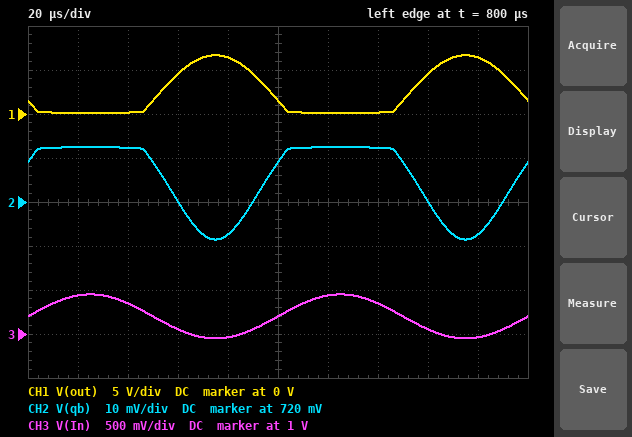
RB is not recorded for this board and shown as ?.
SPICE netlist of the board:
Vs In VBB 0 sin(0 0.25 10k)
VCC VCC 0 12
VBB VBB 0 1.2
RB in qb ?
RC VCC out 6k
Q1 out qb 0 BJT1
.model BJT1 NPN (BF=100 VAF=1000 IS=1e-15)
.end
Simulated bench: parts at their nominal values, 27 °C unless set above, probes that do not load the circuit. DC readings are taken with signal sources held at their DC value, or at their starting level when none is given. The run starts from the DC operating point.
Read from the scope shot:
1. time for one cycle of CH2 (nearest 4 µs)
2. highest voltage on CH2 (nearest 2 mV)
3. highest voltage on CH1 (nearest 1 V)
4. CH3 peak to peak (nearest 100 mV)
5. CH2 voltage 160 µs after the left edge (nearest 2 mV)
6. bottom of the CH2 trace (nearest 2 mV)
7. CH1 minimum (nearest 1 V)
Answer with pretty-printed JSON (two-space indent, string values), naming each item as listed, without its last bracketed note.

{
  "time for one cycle of CH2": "100 µs",
  "highest voltage on CH2": "732 mV",
  "highest voltage on CH1": "7 V",
  "CH3 peak to peak": "500 mV",
  "CH2 voltage 160 µs after the left edge": "720 mV",
  "bottom of the CH2 trace": "712 mV",
  "CH1 minimum": "0 V"
}
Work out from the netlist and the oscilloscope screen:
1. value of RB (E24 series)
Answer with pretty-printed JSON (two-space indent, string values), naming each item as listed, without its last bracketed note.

{
  "value of RB": "27 kΩ"
}
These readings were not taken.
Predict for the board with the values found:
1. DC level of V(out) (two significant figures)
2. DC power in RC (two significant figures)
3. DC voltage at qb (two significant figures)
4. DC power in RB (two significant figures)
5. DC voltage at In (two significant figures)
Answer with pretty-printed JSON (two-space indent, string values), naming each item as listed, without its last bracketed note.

{
  "DC level of V(out)": "1.5 V",
  "DC power in RC": "18 mW",
  "DC voltage at qb": "730 mV",
  "DC power in RB": "8.2 µW",
  "DC voltage at In": "1.2 V"
}
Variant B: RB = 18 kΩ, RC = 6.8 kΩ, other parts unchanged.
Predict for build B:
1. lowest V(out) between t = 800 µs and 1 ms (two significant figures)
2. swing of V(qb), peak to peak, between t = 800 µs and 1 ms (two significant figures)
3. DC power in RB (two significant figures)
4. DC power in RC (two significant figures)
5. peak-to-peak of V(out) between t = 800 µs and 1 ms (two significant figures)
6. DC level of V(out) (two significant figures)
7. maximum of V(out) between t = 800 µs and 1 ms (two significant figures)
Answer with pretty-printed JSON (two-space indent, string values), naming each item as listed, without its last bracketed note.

{
  "lowest V(out) between t = 800 µs and 1 ms": "110 mV",
  "swing of V(qb), peak to peak, between t = 800 µs and 1 ms": "8.9 mV",
  "DC power in RB": "12 µW",
  "DC power in RC": "21 mW",
  "peak-to-peak of V(out) between t = 800 µs and 1 ms": "3.2 V",
  "DC level of V(out)": "140 mV",
  "maximum of V(out) between t = 800 µs and 1 ms": "3.3 V"
}
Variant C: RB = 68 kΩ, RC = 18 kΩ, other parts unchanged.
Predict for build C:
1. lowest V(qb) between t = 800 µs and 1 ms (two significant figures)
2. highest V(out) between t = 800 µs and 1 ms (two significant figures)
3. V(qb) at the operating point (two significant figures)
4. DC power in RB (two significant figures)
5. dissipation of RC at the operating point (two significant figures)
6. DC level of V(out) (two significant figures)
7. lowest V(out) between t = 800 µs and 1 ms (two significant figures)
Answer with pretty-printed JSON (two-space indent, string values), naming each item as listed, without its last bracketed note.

{
  "lowest V(qb) between t = 800 µs and 1 ms": "690 mV",
  "highest V(out) between t = 800 µs and 1 ms": "5.1 V",
  "V(qb) at the operating point": "700 mV",
  "DC power in RB": "3.6 µW",
  "dissipation of RC at the operating point": "7.8 mW",
  "DC level of V(out)": "180 mV",
  "lowest V(out) between t = 800 µs and 1 ms": "130 mV"
}
